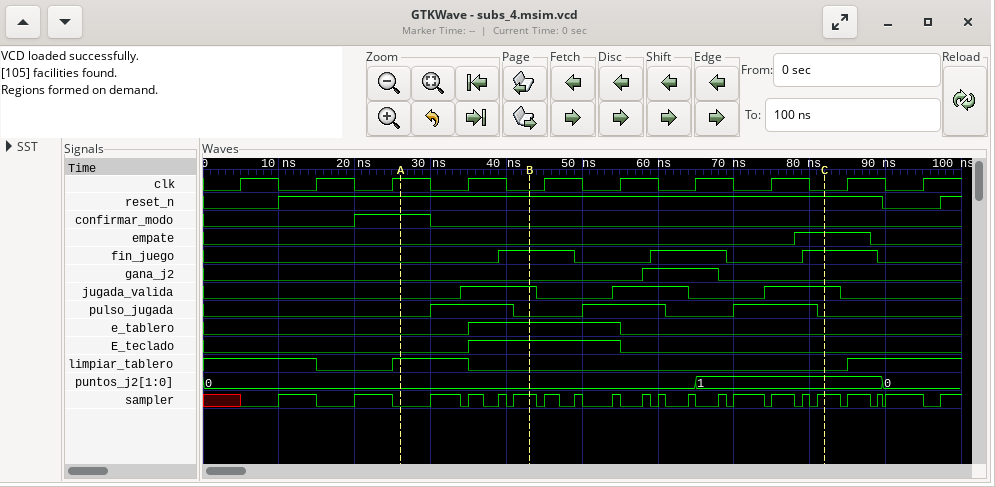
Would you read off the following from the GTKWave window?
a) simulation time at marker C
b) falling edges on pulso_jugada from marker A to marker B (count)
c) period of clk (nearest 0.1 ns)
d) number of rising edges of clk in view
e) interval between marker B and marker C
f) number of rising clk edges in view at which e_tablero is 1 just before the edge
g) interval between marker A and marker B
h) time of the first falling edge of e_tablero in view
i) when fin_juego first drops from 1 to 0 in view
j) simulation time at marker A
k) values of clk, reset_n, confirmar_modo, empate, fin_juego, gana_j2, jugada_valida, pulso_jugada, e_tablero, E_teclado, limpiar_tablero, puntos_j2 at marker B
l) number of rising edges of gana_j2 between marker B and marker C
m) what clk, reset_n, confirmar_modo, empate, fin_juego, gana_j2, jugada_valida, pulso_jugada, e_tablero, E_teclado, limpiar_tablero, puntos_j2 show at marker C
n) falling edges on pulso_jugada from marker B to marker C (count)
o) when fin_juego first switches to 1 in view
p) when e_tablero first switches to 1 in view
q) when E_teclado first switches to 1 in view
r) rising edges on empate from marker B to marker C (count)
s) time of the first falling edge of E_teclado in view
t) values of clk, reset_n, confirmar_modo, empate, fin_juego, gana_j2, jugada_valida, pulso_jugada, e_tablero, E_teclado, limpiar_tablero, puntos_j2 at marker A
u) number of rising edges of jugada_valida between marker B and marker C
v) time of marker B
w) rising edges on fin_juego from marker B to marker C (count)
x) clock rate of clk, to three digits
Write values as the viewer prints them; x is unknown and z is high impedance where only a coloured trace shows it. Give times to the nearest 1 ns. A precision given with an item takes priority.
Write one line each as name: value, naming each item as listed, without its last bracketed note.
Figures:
simulation time at marker C: 82 ns
falling edges on pulso_jugada from marker A to marker B: 1
period of clk: 10 ns
number of rising edges of clk in view: 10
interval between marker B and marker C: 39 ns
number of rising clk edges in view at which e_tablero is 1 just before the edge: 2
interval between marker A and marker B: 17 ns
time of the first falling edge of e_tablero in view: 55 ns
when fin_juego first drops from 1 to 0 in view: 49 ns
simulation time at marker A: 26 ns
values of clk, reset_n, confirmar_modo, empate, fin_juego, gana_j2, jugada_valida, pulso_jugada, e_tablero, E_teclado, limpiar_tablero, puntos_j2 at marker B: clk=0, reset_n=1, confirmar_modo=0, empate=0, fin_juego=1, gana_j2=0, jugada_valida=1, pulso_jugada=0, e_tablero=1, E_teclado=1, limpiar_tablero=0, puntos_j2=0
number of rising edges of gana_j2 between marker B and marker C: 1
what clk, reset_n, confirmar_modo, empate, fin_juego, gana_j2, jugada_valida, pulso_jugada, e_tablero, E_teclado, limpiar_tablero, puntos_j2 show at marker C: clk=0, reset_n=1, confirmar_modo=0, empate=1, fin_juego=1, gana_j2=0, jugada_valida=1, pulso_jugada=0, e_tablero=0, E_teclado=0, limpiar_tablero=0, puntos_j2=1
falling edges on pulso_jugada from marker B to marker C: 2
when fin_juego first switches to 1 in view: 39 ns
when e_tablero first switches to 1 in view: 35 ns
when E_teclado first switches to 1 in view: 35 ns
rising edges on empate from marker B to marker C: 1
time of the first falling edge of E_teclado in view: 55 ns
values of clk, reset_n, confirmar_modo, empate, fin_juego, gana_j2, jugada_valida, pulso_jugada, e_tablero, E_teclado, limpiar_tablero, puntos_j2 at marker A: clk=1, reset_n=1, confirmar_modo=1, empate=0, fin_juego=0, gana_j2=0, jugada_valida=0, pulso_jugada=0, e_tablero=0, E_teclado=0, limpiar_tablero=1, puntos_j2=0
number of rising edges of jugada_valida between marker B and marker C: 2
time of marker B: 43 ns
rising edges on fin_juego from marker B to marker C: 2
clock rate of clk, to three digits: 100 MHz
